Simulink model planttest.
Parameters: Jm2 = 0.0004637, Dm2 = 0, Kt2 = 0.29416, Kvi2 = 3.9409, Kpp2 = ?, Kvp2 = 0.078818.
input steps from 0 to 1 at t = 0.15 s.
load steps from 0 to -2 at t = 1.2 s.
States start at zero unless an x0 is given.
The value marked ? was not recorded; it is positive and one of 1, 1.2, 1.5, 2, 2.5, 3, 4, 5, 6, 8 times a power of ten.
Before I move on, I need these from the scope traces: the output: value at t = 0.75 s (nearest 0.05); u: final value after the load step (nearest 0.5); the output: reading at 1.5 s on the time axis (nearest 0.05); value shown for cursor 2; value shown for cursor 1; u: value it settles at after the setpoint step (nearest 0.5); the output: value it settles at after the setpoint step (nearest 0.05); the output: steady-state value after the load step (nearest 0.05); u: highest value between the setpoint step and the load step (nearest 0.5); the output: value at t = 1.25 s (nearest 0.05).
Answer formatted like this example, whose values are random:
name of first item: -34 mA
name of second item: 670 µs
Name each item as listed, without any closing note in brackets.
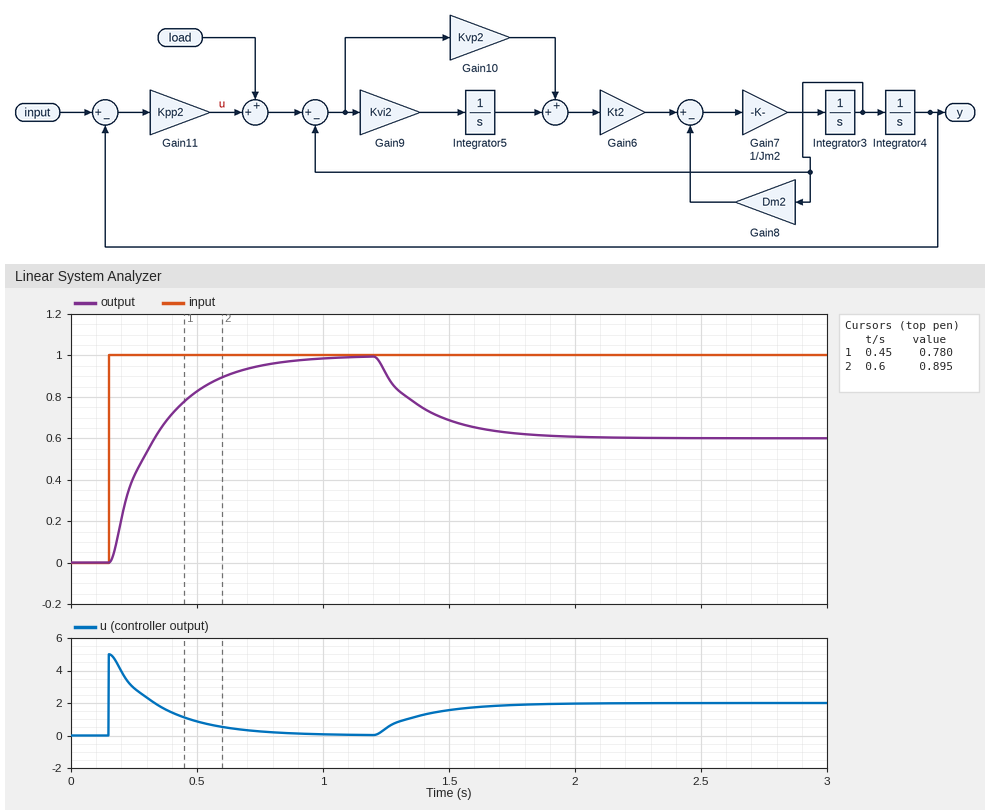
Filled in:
the output: value at t = 0.75 s: 0.95
u: final value after the load step: 2.0
the output: reading at 1.5 s on the time axis: 0.70
value shown for cursor 2: 0.895
value shown for cursor 1: 0.780
u: value it settles at after the setpoint step: 0.0
the output: value it settles at after the setpoint step: 1.00
the output: steady-state value after the load step: 0.60
u: highest value between the setpoint step and the load step: 5.0
the output: value at t = 1.25 s: 0.90
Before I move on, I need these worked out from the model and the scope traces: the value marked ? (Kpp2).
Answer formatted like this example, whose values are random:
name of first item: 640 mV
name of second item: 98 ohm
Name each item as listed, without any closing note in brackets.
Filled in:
the value marked ?: 5
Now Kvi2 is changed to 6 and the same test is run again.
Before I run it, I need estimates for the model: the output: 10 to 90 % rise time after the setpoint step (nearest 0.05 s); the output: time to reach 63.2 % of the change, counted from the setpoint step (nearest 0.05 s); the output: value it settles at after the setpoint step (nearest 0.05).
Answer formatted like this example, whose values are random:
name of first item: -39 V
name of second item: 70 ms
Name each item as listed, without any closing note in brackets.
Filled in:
the output: 10 to 90 % rise time after the setpoint step: 0.45 s
the output: time to reach 63.2 % of the change, counted from the setpoint step: 0.20 s
the output: value it settles at after the setpoint step: 1.00
